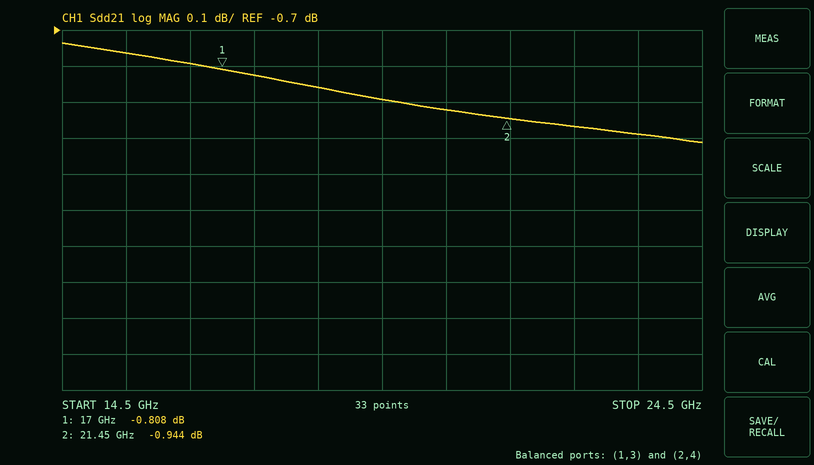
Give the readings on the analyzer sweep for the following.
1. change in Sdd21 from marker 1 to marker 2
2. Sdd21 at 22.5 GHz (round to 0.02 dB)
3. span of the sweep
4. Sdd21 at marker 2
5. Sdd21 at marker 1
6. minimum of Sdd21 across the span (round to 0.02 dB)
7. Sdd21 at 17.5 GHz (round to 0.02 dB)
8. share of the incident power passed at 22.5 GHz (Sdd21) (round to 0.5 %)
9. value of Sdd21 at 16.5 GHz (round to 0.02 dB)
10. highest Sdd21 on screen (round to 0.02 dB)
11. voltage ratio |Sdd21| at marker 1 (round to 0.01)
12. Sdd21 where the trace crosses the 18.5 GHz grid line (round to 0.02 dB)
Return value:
-0.136 dB
-0.96 dB
10 GHz
-0.944 dB
-0.808 dB
-1.02 dB
-0.82 dB
80.0 %
-0.80 dB
-0.74 dB
0.91
-0.86 dB
